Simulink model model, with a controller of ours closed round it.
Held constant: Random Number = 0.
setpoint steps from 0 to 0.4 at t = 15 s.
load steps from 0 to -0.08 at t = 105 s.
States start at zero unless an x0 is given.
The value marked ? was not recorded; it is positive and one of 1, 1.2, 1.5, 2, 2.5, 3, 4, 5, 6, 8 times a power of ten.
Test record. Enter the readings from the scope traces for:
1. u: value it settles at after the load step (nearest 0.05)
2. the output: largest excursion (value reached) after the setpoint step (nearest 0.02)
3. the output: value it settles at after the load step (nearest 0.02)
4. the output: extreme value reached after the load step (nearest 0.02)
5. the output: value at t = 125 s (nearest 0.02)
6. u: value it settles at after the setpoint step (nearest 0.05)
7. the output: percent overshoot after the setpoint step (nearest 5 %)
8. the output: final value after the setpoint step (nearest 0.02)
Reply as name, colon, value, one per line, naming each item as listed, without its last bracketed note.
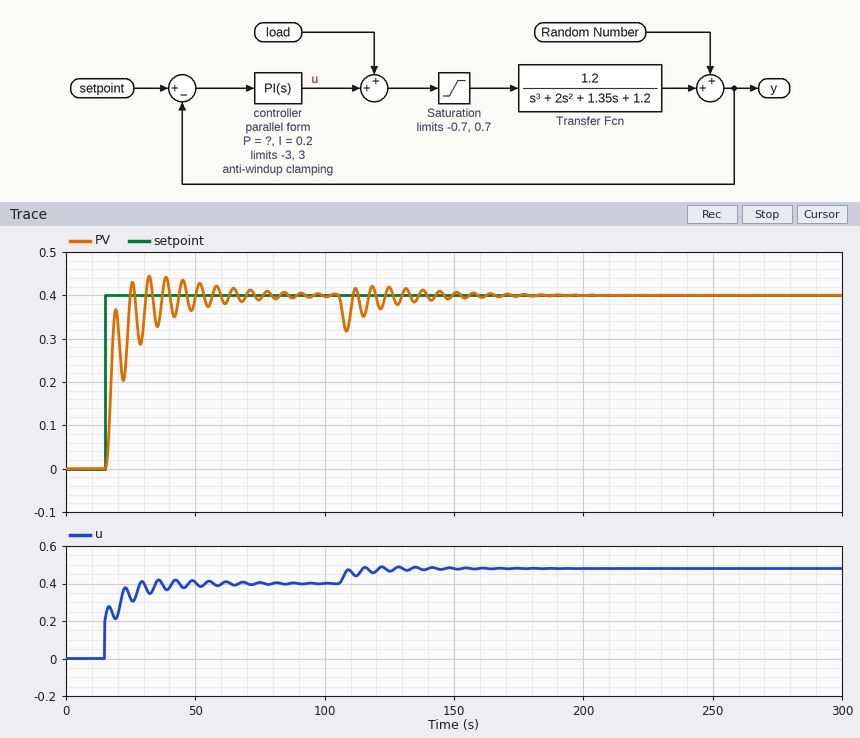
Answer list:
u: value it settles at after the load step: 0.50
the output: largest excursion (value reached) after the setpoint step: 0.44
the output: value it settles at after the load step: 0.40
the output: extreme value reached after the load step: 0.32
the output: value at t = 125 s: 0.42
u: value it settles at after the setpoint step: 0.40
the output: percent overshoot after the setpoint step: 10 %
the output: final value after the setpoint step: 0.40
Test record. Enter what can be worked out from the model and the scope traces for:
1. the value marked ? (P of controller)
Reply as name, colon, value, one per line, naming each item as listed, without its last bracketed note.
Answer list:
the value marked ?: 0.5
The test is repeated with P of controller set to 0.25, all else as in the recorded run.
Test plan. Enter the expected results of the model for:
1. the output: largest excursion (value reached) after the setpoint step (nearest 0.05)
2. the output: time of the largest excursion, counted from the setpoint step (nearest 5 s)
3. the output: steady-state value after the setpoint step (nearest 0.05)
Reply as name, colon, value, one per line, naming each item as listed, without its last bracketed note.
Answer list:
the output: largest excursion (value reached) after the setpoint step: 0.40
the output: time of the largest excursion, counted from the setpoint step: 20 s
the output: steady-state value after the setpoint step: 0.40
